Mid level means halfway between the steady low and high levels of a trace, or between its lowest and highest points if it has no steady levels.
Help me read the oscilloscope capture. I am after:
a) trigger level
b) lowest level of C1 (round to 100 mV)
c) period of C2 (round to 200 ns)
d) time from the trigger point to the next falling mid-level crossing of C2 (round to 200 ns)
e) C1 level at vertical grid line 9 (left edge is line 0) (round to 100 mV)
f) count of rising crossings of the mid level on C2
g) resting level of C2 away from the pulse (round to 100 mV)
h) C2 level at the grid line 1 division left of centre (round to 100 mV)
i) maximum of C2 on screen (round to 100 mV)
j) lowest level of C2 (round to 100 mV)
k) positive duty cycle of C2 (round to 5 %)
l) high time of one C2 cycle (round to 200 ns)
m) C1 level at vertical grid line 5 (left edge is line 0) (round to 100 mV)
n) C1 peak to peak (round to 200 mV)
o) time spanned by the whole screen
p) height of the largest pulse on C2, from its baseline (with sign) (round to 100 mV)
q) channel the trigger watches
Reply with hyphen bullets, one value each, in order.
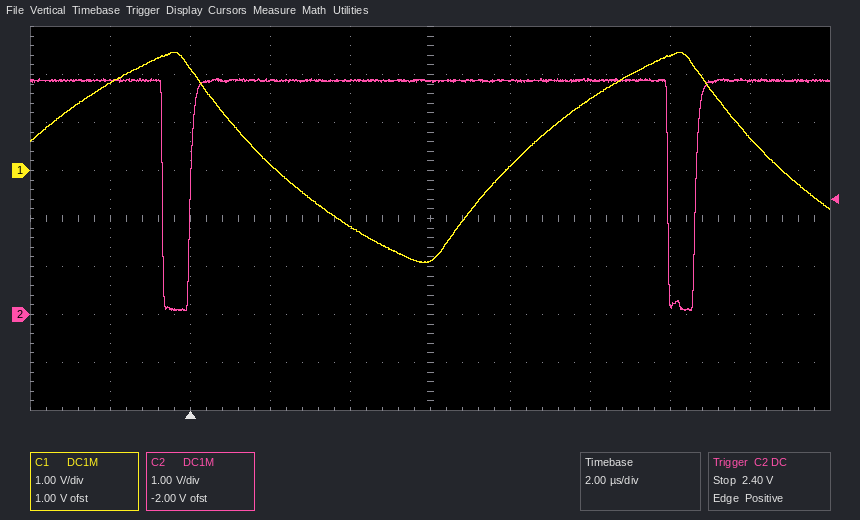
- 2.40 V
- -1.9 V
- 12.6 µs
- 12.0 µs
- 700 mV
- 2
- 4.9 V
- 4.9 V
- 4.9 V
- 100 mV
- 95 %
- 12.0 µs
- -1.9 V
- 4.4 V
- 20 µs
- -4.8 V
- C2
